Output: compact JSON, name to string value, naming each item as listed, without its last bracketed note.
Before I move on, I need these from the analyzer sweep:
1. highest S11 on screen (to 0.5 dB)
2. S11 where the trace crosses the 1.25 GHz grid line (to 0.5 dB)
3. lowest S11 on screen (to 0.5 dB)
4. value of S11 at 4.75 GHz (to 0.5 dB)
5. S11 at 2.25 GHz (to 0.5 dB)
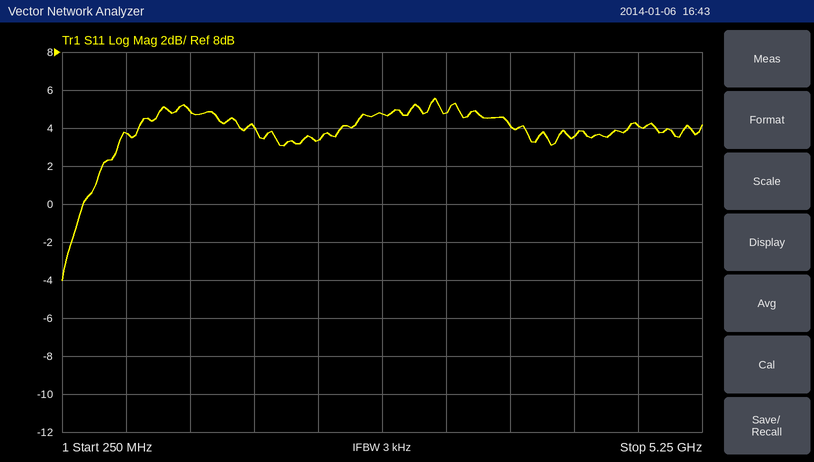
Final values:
{"highest S11 on screen": "5.5 dB", "S11 where the trace crosses the 1.25 GHz grid line": "5.0 dB", "lowest S11 on screen": "-4.0 dB", "value of S11 at 4.75 GHz": "4.0 dB", "S11 at 2.25 GHz": "3.5 dB"}
